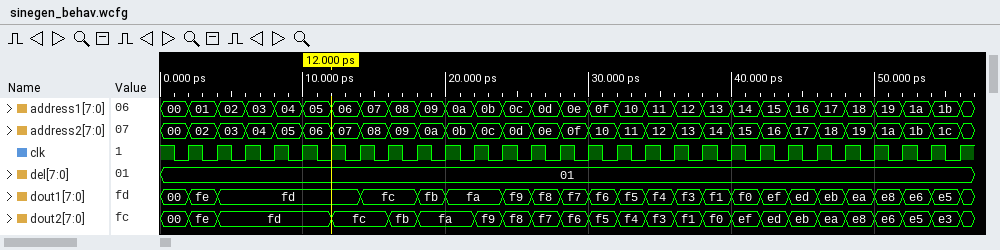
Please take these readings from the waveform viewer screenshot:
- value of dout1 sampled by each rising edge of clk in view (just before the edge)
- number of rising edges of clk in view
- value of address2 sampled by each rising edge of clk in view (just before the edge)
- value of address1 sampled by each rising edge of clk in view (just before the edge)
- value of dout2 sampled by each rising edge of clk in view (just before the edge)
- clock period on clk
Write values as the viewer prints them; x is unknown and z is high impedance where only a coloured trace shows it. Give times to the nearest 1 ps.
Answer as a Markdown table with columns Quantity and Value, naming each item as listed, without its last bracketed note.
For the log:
| Quantity | Value |
|---|---|
| value of dout1 sampled by each rising edge of clk in view | 00, fe, fd, fd, fd, fd, fd, fc, fc, fb, fa, fa, f9, f8, f7, f6, f5, f4, f3, f1, f0, ef, ed, eb, ea, e8, e6, e5 |
| number of rising edges of clk in view | 28 |
| value of address2 sampled by each rising edge of clk in view | 00, 02, 03, 04, 05, 06, 07, 08, 09, 0a, 0b, 0c, 0d, 0e, 0f, 10, 11, 12, 13, 14, 15, 16, 17, 18, 19, 1a, 1b, 1c |
| value of address1 sampled by each rising edge of clk in view | 00, 01, 02, 03, 04, 05, 06, 07, 08, 09, 0a, 0b, 0c, 0d, 0e, 0f, 10, 11, 12, 13, 14, 15, 16, 17, 18, 19, 1a, 1b |
| value of dout2 sampled by each rising edge of clk in view | 00, fe, fd, fd, fd, fd, fc, fc, fb, fa, fa, f9, f8, f7, f6, f5, f4, f3, f1, f0, ef, ed, eb, ea, e8, e6, e5, e3 |
| clock period on clk | 2 ps |
